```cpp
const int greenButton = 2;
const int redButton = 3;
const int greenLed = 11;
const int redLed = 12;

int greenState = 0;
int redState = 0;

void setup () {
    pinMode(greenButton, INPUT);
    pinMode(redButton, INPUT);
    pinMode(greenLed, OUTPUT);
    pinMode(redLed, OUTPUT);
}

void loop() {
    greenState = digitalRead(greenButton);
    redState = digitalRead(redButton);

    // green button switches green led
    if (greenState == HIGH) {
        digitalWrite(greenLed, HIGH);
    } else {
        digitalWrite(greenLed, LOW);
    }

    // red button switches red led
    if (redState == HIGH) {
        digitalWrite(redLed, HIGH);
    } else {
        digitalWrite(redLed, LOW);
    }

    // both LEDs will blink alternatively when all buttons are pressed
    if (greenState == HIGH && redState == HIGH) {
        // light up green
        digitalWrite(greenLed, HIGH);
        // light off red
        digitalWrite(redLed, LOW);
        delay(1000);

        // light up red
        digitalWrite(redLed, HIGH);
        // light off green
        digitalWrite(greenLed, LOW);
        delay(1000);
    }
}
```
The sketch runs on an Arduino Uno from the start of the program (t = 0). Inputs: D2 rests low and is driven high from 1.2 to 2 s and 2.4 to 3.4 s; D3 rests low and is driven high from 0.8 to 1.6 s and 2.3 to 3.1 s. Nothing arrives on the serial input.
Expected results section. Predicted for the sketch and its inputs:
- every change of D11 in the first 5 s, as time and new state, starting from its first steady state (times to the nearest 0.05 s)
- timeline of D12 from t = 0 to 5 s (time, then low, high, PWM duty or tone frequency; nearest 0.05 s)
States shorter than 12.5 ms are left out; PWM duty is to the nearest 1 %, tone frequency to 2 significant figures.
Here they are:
0 s low; 1.2 s high; 2.2 s low; 3.2 s high; 3.4 s low
0 s low; 0.8 s high; 1.2 s low; 2.2 s high; 3.2 s low
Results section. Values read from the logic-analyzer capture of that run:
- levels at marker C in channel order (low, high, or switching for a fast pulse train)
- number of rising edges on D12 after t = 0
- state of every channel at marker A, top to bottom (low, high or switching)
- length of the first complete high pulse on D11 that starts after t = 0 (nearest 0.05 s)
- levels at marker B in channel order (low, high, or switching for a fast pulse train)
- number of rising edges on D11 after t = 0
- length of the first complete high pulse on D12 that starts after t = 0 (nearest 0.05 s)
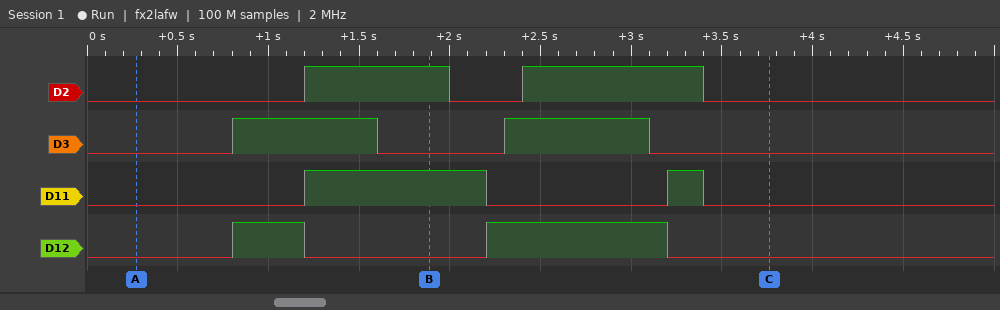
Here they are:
D2 low, D3 low, D11 low, D12 low
2
D2 low, D3 low, D11 low, D12 low
1.00 s
D2 high, D3 low, D11 high, D12 low
2
0.40 s
